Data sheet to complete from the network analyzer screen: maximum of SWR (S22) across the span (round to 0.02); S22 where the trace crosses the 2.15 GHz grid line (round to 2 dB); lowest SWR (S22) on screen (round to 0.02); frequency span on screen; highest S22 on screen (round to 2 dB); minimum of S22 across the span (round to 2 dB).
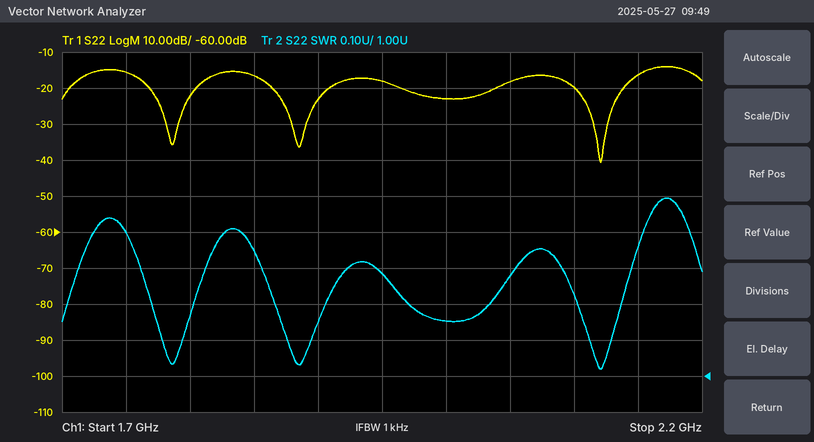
1.50
-16 dB
1.02
500 MHz
-14 dB
-40 dB
